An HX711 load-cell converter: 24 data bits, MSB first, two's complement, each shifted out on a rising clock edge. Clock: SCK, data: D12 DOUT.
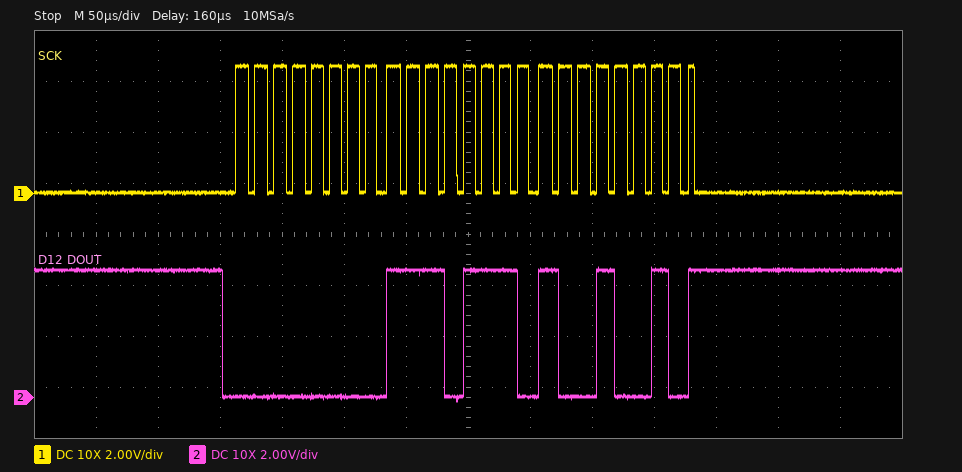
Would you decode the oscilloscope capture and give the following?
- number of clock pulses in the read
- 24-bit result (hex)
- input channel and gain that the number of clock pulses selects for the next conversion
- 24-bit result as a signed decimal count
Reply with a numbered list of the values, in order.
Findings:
1. 25
2. 0x00EE92
3. channel A, gain 128
4. 61074
